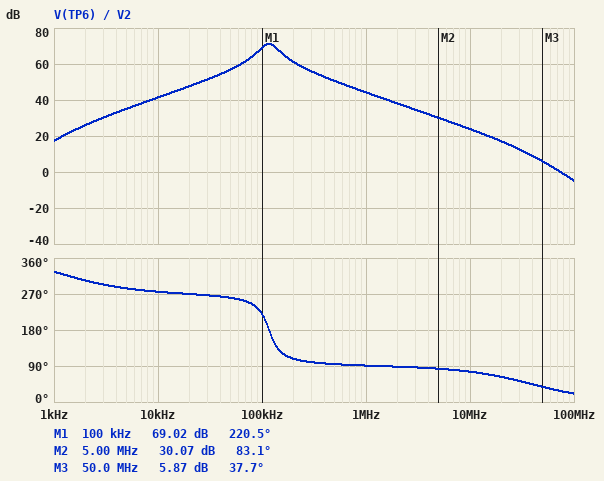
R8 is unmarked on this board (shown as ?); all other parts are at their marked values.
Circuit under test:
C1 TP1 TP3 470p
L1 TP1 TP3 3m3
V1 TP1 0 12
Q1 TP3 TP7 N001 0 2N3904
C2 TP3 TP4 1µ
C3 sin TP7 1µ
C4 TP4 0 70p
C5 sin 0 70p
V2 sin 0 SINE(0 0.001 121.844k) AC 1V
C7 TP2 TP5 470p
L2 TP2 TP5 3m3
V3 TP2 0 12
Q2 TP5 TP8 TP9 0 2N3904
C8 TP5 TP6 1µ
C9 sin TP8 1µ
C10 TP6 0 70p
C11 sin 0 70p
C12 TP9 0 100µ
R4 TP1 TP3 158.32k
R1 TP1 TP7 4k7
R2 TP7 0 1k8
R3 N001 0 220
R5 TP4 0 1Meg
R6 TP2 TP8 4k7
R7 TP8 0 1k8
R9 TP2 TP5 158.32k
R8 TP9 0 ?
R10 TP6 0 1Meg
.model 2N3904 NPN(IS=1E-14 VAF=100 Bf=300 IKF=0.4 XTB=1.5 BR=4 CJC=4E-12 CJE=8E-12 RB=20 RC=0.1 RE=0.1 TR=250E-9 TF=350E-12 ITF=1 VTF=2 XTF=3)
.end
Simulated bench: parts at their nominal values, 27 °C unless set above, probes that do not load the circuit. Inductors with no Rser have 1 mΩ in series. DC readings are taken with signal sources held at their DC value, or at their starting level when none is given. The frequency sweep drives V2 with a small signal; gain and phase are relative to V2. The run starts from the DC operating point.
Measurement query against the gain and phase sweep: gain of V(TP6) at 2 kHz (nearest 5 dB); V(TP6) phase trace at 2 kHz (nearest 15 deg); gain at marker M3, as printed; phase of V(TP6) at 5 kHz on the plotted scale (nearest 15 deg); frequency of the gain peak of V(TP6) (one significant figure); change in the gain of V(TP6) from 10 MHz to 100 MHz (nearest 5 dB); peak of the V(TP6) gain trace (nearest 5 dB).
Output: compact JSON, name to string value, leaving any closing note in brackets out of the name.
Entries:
{"gain of V(TP6) at 2 kHz": "25 dB", "V(TP6) phase trace at 2 kHz": "300 deg", "gain at marker M3, as printed": "5.87 dB", "phase of V(TP6) at 5 kHz on the plotted scale": "285 deg", "frequency of the gain peak of V(TP6)": "100 kHz", "change in the gain of V(TP6) from 10 MHz to 100 MHz": "-30 dB", "peak of the V(TP6) gain trace": "70 dB"}
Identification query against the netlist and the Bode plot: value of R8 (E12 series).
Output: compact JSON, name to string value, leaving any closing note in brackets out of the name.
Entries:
{"value of R8": "150 Ω"}
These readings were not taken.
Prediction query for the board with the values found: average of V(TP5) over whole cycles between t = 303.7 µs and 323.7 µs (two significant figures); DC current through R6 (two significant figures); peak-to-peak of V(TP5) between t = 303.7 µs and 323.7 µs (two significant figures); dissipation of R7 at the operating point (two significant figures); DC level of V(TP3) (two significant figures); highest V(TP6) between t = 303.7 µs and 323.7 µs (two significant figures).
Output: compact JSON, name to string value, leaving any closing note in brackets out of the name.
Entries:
{"average of V(TP5) over whole cycles between t = 303.7 µs and 323.7 µs": "12 V", "DC current through R6": "1.9 mA", "peak-to-peak of V(TP5) between t = 303.7 µs and 323.7 µs": "7.2 V", "dissipation of R7 at the operating point": "5.9 mW", "DC level of V(TP3)": "12 V", "highest V(TP6) between t = 303.7 µs and 323.7 µs": "3.6 V"}
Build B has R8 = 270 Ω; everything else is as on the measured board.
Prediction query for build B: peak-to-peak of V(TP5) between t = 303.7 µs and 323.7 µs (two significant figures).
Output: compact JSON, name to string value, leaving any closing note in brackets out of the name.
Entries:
{"peak-to-peak of V(TP5) between t = 303.7 µs and 323.7 µs": "7.0 V"}
